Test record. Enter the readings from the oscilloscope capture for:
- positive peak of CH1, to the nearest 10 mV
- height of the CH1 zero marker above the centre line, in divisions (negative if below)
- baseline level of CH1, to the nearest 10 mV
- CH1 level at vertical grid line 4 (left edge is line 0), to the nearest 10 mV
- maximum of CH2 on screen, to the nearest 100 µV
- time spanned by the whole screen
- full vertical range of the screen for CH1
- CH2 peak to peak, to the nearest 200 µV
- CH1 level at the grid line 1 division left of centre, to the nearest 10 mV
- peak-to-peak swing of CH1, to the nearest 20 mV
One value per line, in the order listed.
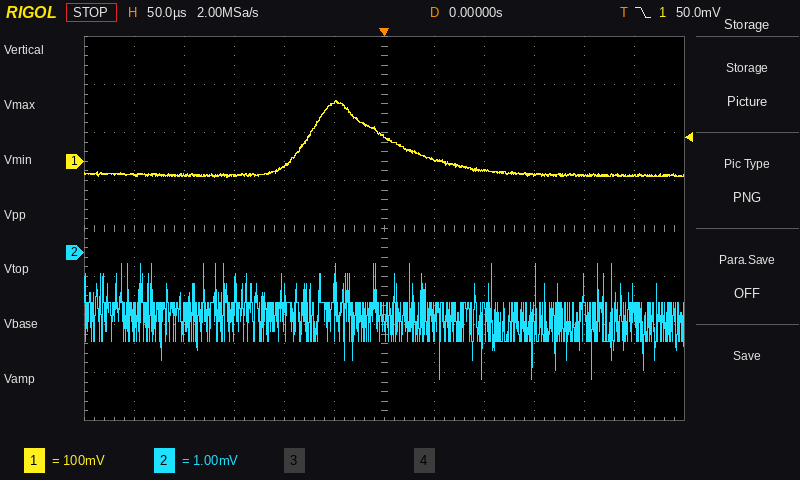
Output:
130 mV
+1.4 div
-30 mV
-10 mV
-200 µV
600 µs
800 mV
2.4 mV
120 mV
160 mV
